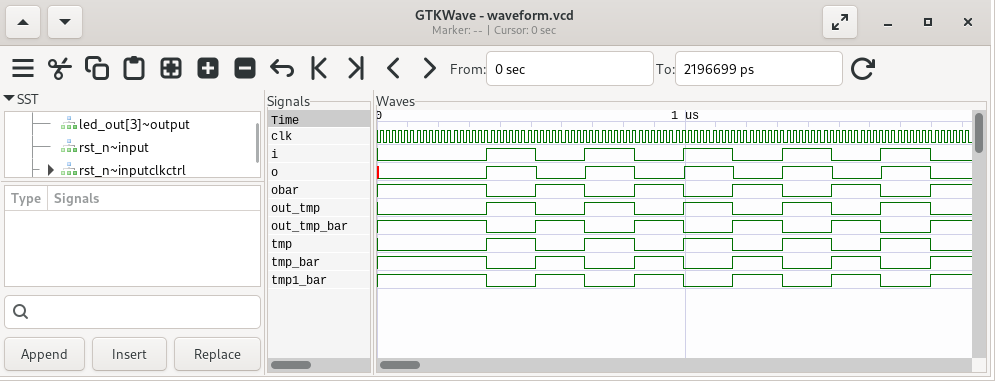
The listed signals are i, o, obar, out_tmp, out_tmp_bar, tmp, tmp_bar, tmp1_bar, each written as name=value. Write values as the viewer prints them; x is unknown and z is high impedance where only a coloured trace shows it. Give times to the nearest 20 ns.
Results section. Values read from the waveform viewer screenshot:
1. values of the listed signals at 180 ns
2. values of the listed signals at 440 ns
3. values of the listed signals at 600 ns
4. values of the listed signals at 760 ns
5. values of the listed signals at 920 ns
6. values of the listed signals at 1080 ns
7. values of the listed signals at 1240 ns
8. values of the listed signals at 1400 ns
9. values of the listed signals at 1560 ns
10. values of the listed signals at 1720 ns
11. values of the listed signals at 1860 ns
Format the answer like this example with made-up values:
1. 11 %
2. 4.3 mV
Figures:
1. i=0, o=0, obar=1, out_tmp=0, out_tmp_bar=1, tmp=0, tmp_bar=1, tmp1_bar=1
2. i=1, o=1, obar=0, out_tmp=1, out_tmp_bar=0, tmp=1, tmp_bar=0, tmp1_bar=0
3. i=0, o=0, obar=1, out_tmp=0, out_tmp_bar=1, tmp=0, tmp_bar=1, tmp1_bar=1
4. i=1, o=1, obar=0, out_tmp=1, out_tmp_bar=0, tmp=1, tmp_bar=0, tmp1_bar=0
5. i=0, o=0, obar=1, out_tmp=0, out_tmp_bar=1, tmp=0, tmp_bar=1, tmp1_bar=1
6. i=1, o=1, obar=0, out_tmp=1, out_tmp_bar=0, tmp=1, tmp_bar=0, tmp1_bar=0
7. i=0, o=0, obar=1, out_tmp=0, out_tmp_bar=1, tmp=0, tmp_bar=1, tmp1_bar=1
8. i=1, o=1, obar=0, out_tmp=1, out_tmp_bar=0, tmp=1, tmp_bar=0, tmp1_bar=0
9. i=0, o=0, obar=1, out_tmp=0, out_tmp_bar=1, tmp=0, tmp_bar=1, tmp1_bar=1
10. i=1, o=1, obar=0, out_tmp=1, out_tmp_bar=0, tmp=1, tmp_bar=0, tmp1_bar=0
11. i=0, o=0, obar=1, out_tmp=0, out_tmp_bar=1, tmp=0, tmp_bar=1, tmp1_bar=1
